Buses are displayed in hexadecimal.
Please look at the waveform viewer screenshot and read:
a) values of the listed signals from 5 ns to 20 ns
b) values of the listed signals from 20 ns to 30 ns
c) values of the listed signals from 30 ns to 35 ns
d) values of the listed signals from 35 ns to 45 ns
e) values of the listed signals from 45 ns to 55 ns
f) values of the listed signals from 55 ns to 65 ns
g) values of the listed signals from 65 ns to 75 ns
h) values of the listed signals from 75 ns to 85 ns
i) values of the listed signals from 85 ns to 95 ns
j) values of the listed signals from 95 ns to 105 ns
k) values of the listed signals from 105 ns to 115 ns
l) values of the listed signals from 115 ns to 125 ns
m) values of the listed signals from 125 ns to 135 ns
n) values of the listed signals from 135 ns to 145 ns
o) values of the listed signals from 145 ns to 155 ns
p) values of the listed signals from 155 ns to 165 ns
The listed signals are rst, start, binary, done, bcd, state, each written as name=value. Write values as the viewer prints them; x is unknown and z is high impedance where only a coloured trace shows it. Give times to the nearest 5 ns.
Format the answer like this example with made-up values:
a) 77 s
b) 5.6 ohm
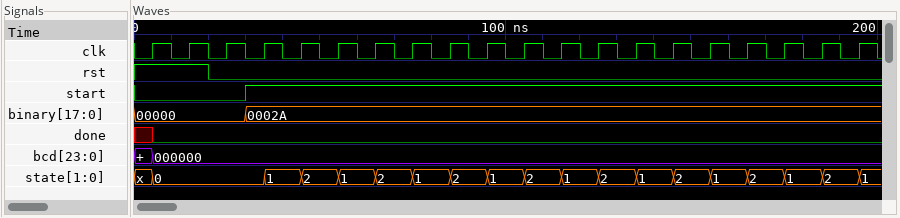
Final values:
a) rst=1, start=0, binary=00000, done=0, bcd=000000, state=0
b) rst=0, start=0, binary=00000, done=0, bcd=000000, state=0
c) rst=0, start=1, binary=0002A, done=0, bcd=000000, state=0
d) rst=0, start=1, binary=0002A, done=0, bcd=000000, state=1
e) rst=0, start=1, binary=0002A, done=0, bcd=000000, state=2
f) rst=0, start=1, binary=0002A, done=0, bcd=000000, state=1
g) rst=0, start=1, binary=0002A, done=0, bcd=000000, state=2
h) rst=0, start=1, binary=0002A, done=0, bcd=000000, state=1
i) rst=0, start=1, binary=0002A, done=0, bcd=000000, state=2
j) rst=0, start=1, binary=0002A, done=0, bcd=000000, state=1
k) rst=0, start=1, binary=0002A, done=0, bcd=000000, state=2
l) rst=0, start=1, binary=0002A, done=0, bcd=000000, state=1
m) rst=0, start=1, binary=0002A, done=0, bcd=000000, state=2
n) rst=0, start=1, binary=0002A, done=0, bcd=000000, state=1
o) rst=0, start=1, binary=0002A, done=0, bcd=000000, state=2
p) rst=0, start=1, binary=0002A, done=0, bcd=000000, state=1
